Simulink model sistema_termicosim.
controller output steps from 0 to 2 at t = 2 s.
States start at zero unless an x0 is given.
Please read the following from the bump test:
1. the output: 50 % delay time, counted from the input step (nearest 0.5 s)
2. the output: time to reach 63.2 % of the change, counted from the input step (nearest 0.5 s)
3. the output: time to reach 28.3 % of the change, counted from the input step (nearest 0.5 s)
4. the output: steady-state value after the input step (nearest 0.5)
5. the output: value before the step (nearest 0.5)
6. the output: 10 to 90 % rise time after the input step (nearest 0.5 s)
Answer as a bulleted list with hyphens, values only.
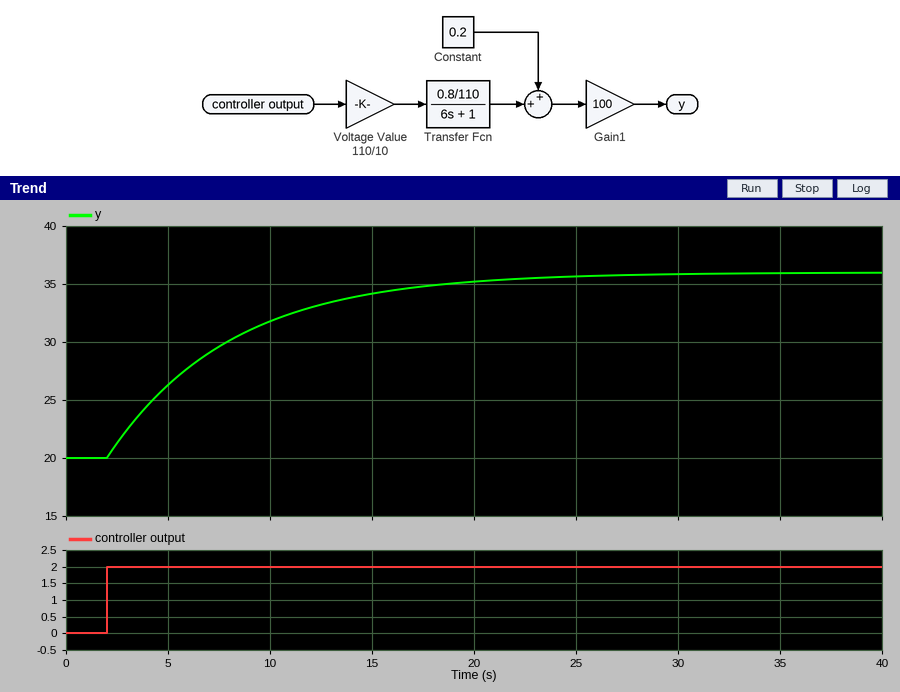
- 4.0 s
- 6.0 s
- 2.0 s
- 36.0
- 20.0
- 13.0 s
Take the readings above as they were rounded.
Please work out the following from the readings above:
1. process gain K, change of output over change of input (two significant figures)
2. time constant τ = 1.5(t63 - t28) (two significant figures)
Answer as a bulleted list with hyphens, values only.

- 8.0
- 6.0 s
